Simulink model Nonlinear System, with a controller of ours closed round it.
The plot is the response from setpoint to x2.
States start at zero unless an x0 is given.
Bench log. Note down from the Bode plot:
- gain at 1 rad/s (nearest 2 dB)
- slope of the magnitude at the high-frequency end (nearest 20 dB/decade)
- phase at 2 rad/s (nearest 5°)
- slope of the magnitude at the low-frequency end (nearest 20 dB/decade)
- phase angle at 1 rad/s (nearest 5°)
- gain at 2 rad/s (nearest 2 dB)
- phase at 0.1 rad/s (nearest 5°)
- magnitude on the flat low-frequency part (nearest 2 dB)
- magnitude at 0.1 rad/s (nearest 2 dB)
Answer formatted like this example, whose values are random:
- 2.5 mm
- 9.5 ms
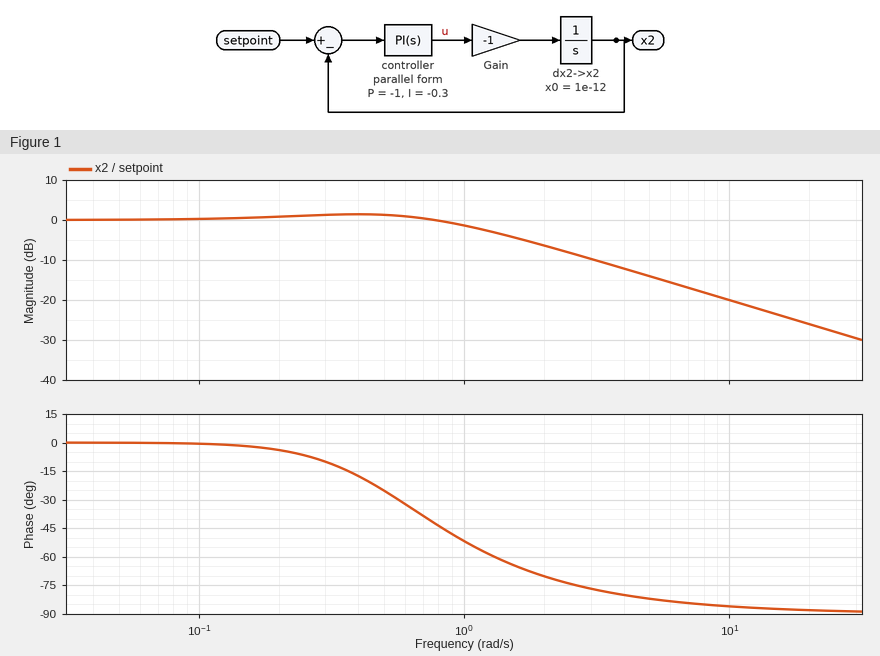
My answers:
- -2 dB
- -20 dB/decade
- -70°
- 0 dB/decade
- -50°
- -6 dB
- 0°
- 0 dB
- 0 dB
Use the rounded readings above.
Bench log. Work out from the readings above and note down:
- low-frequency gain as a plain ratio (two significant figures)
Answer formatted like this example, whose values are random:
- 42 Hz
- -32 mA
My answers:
- 1.0
